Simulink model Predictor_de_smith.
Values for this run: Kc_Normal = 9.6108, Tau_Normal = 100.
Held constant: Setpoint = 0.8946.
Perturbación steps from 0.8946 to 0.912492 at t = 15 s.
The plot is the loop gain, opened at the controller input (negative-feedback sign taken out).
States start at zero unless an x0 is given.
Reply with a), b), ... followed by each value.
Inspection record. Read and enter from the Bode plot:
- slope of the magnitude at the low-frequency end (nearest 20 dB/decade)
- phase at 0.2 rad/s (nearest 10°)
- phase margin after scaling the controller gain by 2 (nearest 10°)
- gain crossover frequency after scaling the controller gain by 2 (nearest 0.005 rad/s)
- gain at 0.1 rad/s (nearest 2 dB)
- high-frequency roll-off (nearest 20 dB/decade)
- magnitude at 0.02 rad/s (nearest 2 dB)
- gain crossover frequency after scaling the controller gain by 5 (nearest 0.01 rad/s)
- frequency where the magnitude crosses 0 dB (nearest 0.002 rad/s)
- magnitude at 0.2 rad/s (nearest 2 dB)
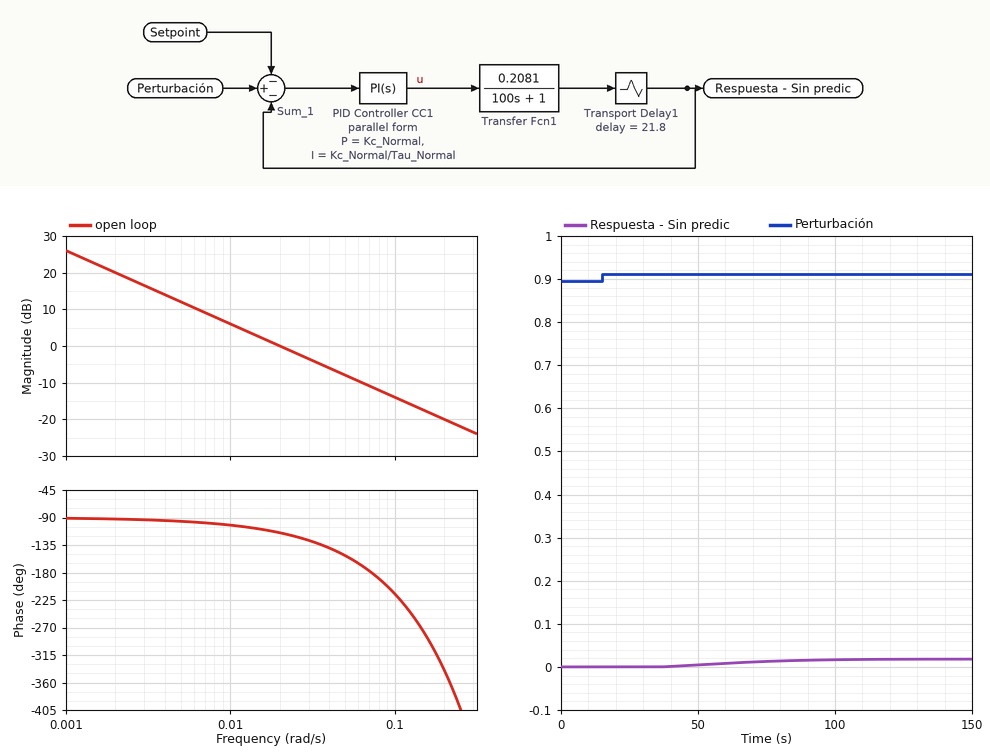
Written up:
a) -20 dB/decade
b) -340°
c) 40°
d) 0.040 rad/s
e) -14 dB
f) -20 dB/decade
g) 0 dB
h) 0.10 rad/s
i) 0.020 rad/s
j) -20 dB
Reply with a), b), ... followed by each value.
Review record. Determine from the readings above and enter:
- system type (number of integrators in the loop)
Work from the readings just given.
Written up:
a) 1
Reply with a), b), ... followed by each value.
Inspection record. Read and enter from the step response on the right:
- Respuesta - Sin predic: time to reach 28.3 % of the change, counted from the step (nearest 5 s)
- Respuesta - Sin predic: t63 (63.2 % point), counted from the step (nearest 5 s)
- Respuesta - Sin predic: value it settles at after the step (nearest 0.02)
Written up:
a) 35 s
b) 55 s
c) 0.02
